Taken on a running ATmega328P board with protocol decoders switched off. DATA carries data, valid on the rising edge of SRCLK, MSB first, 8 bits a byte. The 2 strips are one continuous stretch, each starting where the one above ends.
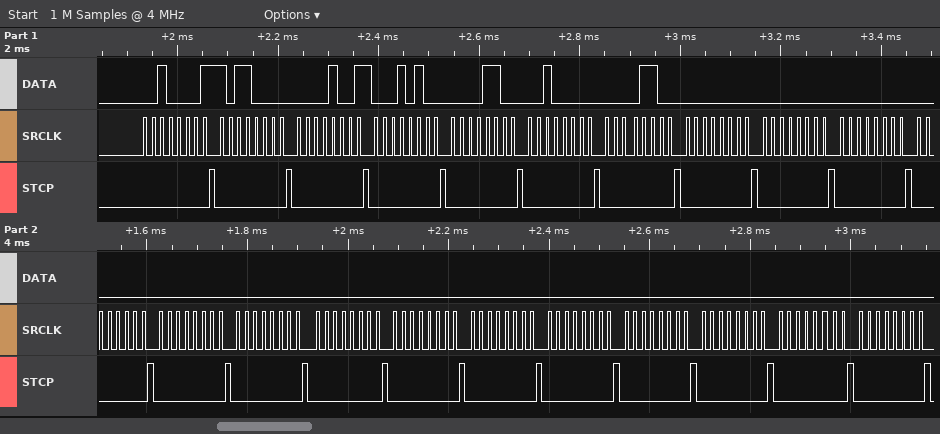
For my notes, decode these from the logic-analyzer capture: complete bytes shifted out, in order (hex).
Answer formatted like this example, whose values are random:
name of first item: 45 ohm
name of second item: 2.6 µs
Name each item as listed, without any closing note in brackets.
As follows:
complete bytes shifted out, in order: 0x21 0xB0 0x09 0x14 0x0C 0x20 0x0C 0x00 0x00 0x00 0x00 0x00 0x00 0x00 0x00 0x00 0x00 0x00 0x00 0x00 0x00
